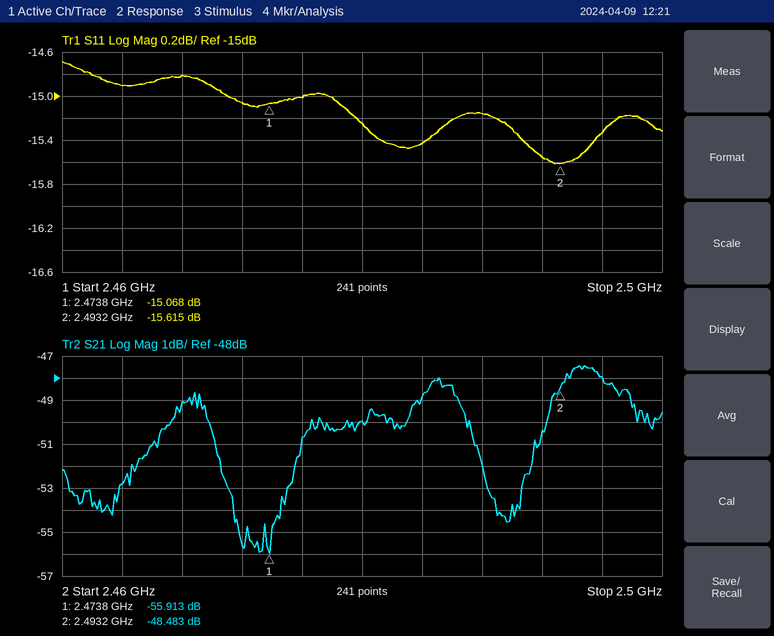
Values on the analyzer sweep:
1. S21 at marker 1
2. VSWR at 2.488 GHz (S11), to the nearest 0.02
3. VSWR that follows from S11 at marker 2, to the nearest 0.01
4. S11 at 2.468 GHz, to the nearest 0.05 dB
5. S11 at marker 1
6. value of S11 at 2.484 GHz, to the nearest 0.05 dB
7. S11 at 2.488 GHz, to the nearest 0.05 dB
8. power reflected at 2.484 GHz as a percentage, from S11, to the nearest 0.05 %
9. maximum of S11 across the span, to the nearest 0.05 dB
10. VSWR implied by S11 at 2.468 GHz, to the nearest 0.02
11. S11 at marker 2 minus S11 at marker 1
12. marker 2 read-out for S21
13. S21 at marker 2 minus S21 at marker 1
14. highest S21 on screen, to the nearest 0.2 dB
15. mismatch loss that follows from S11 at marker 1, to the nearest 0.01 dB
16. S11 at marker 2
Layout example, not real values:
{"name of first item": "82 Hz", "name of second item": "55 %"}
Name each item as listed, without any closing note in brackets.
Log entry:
{"S21 at marker 1": "-55.913 dB", "VSWR at 2.488 GHz (S11), to the nearest 0.02": "1.42", "VSWR that follows from S11 at marker 2, to the nearest 0.01": "1.40", "S11 at 2.468 GHz, to the nearest 0.05 dB": "-14.80 dB", "S11 at marker 1": "-15.068 dB", "value of S11 at 2.484 GHz, to the nearest 0.05 dB": "-15.45 dB", "S11 at 2.488 GHz, to the nearest 0.05 dB": "-15.15 dB", "power reflected at 2.484 GHz as a percentage, from S11, to the nearest 0.05 %": "2.85 %", "maximum of S11 across the span, to the nearest 0.05 dB": "-14.70 dB", "VSWR implied by S11 at 2.468 GHz, to the nearest 0.02": "1.44", "S11 at marker 2 minus S11 at marker 1": "-0.547 dB", "marker 2 read-out for S21": "-48.483 dB", "S21 at marker 2 minus S21 at marker 1": "7.430 dB", "highest S21 on screen, to the nearest 0.2 dB": "-47.4 dB", "mismatch loss that follows from S11 at marker 1, to the nearest 0.01 dB": "0.14 dB", "S11 at marker 2": "-15.615 dB"}
